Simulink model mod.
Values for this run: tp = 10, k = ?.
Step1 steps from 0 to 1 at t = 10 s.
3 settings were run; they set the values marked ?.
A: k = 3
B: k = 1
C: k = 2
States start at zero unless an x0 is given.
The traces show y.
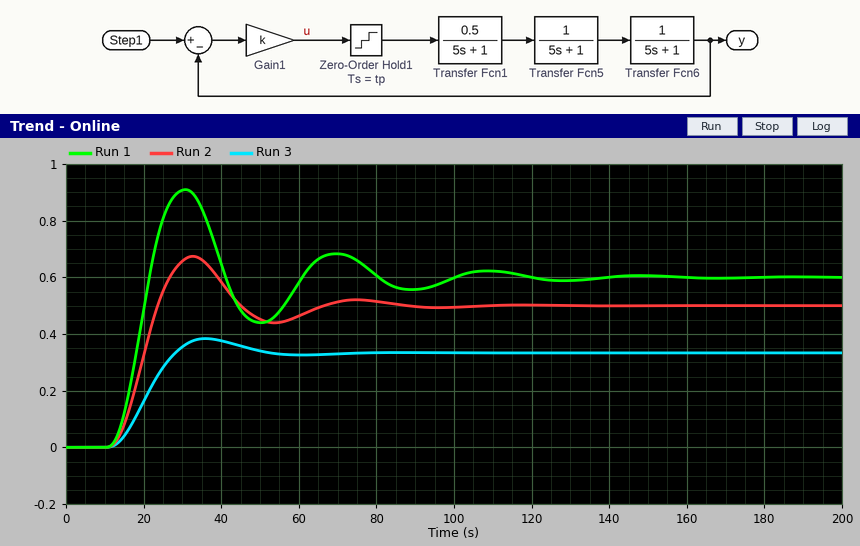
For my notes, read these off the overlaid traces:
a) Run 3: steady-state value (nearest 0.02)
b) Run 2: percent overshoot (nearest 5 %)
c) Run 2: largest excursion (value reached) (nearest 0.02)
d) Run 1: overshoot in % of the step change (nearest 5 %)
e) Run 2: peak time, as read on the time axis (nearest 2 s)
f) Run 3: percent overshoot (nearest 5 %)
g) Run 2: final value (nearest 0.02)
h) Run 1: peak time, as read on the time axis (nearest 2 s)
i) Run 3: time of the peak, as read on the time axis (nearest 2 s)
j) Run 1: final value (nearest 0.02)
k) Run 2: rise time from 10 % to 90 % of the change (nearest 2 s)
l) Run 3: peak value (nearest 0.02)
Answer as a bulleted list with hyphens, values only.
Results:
- 0.34
- 35 %
- 0.68
- 50 %
- 32 s
- 15 %
- 0.50
- 30 s
- 36 s
- 0.60
- 8 s
- 0.38
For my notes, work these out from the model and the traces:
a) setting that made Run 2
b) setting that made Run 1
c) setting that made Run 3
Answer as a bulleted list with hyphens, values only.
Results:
- C
- A
- B
